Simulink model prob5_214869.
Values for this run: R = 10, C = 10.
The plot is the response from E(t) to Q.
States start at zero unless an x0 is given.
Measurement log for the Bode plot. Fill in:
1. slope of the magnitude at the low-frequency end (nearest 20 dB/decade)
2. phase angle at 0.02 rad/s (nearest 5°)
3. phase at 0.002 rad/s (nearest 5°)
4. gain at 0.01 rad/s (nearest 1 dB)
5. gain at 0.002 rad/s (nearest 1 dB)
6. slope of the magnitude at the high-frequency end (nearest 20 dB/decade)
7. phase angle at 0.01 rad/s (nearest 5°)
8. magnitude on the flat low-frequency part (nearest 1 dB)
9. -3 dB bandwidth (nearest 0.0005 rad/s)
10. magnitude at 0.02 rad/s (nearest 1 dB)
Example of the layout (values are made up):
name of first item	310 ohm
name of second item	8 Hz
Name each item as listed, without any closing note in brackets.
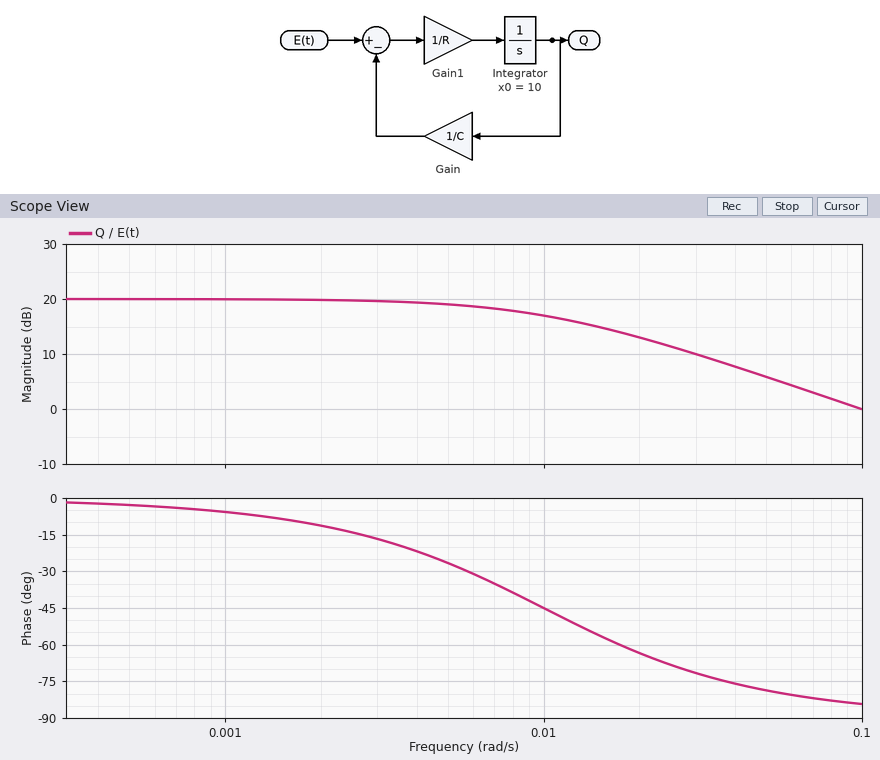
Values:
slope of the magnitude at the low-frequency end	0 dB/decade
phase angle at 0.02 rad/s	-65°
phase at 0.002 rad/s	-10°
gain at 0.01 rad/s	17 dB
gain at 0.002 rad/s	20 dB
slope of the magnitude at the high-frequency end	-20 dB/decade
phase angle at 0.01 rad/s	-45°
magnitude on the flat low-frequency part	20 dB
-3 dB bandwidth	0.0100 rad/s
magnitude at 0.02 rad/s	13 dB
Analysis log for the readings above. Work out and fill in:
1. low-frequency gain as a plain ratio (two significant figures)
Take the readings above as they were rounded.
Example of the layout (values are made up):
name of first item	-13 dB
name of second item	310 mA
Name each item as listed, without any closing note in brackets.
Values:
low-frequency gain as a plain ratio	10
